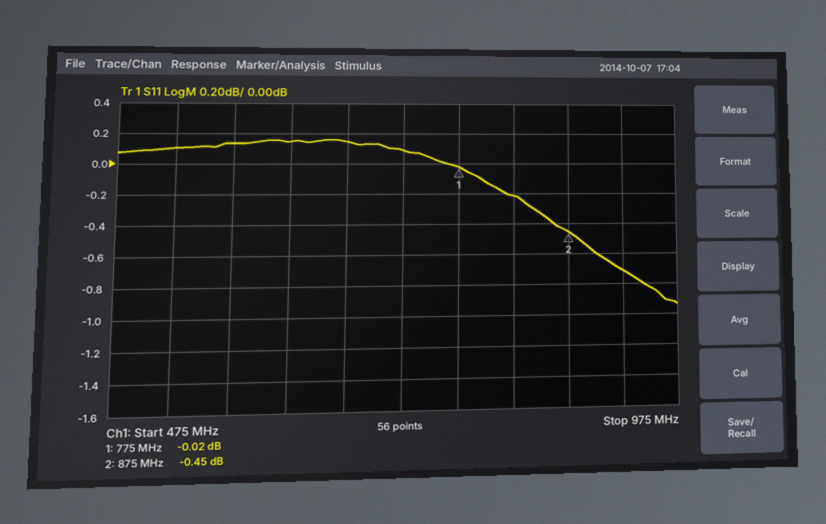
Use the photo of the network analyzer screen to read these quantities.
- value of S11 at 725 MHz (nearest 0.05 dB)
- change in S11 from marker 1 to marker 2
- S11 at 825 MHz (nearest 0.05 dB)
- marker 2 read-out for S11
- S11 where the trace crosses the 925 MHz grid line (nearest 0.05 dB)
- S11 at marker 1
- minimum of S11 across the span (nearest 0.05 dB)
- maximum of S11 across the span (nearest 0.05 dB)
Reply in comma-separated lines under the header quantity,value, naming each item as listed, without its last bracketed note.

quantity,value
value of S11 at 725 MHz,0.10 dB
change in S11 from marker 1 to marker 2,-0.43 dB
S11 at 825 MHz,-0.20 dB
marker 2 read-out for S11,-0.45 dB
S11 where the trace crosses the 925 MHz grid line,-0.70 dB
S11 at marker 1,-0.02 dB
minimum of S11 across the span,-0.95 dB
maximum of S11 across the span,0.15 dB
